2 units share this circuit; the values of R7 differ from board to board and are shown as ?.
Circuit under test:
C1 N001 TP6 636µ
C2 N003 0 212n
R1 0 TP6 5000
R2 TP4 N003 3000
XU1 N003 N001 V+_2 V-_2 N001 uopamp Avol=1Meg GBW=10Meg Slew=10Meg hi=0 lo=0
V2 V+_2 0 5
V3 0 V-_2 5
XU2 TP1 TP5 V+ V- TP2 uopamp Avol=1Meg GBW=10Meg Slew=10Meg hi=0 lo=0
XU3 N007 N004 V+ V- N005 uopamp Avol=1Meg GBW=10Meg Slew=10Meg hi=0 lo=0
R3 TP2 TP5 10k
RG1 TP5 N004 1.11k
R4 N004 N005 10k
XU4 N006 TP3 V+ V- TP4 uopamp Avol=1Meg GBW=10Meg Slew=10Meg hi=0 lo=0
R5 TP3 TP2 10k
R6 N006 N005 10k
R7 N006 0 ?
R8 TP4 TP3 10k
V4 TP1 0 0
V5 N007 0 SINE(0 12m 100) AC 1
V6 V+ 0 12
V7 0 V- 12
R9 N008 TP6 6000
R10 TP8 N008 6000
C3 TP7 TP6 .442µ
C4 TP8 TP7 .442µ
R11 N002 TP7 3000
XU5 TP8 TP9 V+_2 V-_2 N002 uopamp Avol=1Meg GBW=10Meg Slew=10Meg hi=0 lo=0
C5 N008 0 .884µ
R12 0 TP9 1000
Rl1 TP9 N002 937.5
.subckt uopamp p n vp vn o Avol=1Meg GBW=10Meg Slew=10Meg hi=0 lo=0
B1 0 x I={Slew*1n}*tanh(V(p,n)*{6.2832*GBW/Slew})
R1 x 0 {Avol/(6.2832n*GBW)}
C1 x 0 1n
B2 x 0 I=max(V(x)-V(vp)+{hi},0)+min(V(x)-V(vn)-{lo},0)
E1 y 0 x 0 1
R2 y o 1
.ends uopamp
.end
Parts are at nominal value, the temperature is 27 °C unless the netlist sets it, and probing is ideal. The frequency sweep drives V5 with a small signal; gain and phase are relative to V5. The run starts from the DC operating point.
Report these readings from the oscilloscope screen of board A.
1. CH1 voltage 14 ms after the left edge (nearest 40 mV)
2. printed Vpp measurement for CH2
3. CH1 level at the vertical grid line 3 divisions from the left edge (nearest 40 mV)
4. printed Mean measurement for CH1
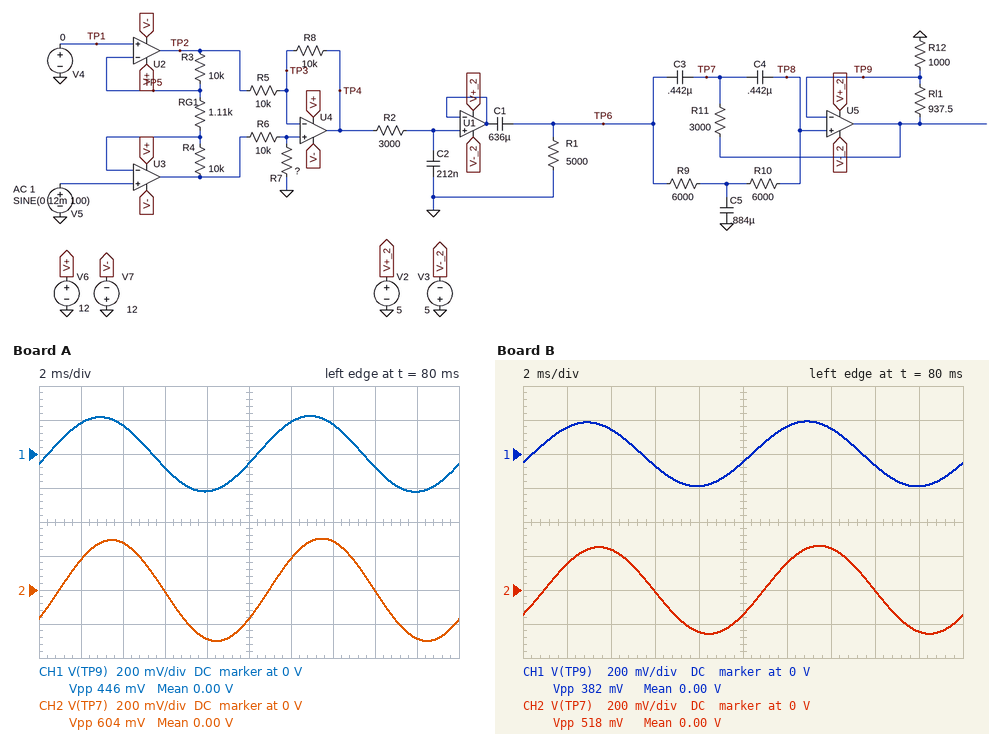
160 mV
604 mV
-80 mV
0.00 V
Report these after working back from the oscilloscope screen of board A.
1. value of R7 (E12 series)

12 kΩ
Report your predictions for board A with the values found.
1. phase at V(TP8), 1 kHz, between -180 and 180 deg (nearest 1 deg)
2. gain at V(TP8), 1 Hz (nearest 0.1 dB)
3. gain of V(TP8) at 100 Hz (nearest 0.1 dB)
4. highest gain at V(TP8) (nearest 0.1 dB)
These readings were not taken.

-76 deg
26.0 dB
25.3 dB
26.0 dB
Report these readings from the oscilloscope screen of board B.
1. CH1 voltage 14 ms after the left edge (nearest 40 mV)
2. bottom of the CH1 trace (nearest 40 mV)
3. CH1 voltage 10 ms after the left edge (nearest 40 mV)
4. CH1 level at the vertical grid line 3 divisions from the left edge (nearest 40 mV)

160 mV
-200 mV
-40 mV
-80 mV
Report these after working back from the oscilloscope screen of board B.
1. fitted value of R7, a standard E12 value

6.8 kΩ
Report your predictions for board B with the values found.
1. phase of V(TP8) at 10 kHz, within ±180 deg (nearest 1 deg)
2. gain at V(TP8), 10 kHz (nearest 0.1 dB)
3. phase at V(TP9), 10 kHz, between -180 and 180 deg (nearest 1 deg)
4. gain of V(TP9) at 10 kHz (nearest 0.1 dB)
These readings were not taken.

-90 deg
-7.4 dB
-90 deg
-7.4 dB
